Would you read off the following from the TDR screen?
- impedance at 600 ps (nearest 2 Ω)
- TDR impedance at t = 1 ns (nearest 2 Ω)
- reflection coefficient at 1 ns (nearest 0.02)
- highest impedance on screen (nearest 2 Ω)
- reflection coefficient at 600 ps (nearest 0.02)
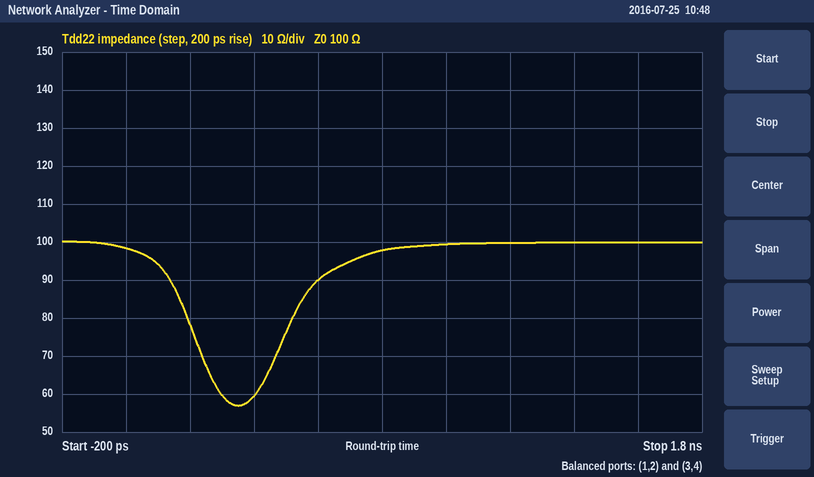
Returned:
90 Ω
100 Ω
0.00
100 Ω
-0.06
